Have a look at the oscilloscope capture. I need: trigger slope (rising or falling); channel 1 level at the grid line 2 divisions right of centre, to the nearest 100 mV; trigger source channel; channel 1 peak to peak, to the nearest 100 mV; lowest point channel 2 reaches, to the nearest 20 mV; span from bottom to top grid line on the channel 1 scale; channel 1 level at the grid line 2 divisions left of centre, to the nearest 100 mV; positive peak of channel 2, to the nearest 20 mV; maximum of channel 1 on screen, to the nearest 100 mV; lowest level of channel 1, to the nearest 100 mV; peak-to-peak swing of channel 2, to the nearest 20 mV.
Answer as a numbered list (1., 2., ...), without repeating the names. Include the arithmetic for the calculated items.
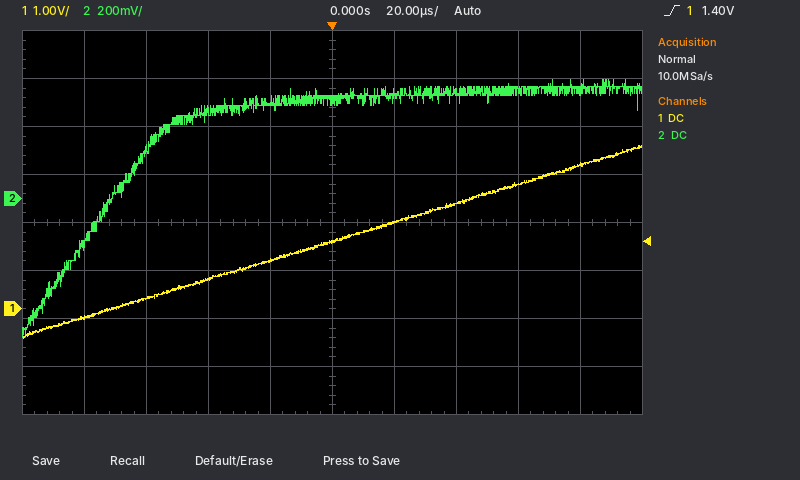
1. rising
2. 2.2 V
3. channel 1
4. 3.4 V − (-600 mV) = 4.0 V
5. -580 mV
6. 8 V
7. 600 mV
8. 500 mV
9. 3.4 V
10. -600 mV
11. 500 mV − (-580 mV) = 1.08 V
